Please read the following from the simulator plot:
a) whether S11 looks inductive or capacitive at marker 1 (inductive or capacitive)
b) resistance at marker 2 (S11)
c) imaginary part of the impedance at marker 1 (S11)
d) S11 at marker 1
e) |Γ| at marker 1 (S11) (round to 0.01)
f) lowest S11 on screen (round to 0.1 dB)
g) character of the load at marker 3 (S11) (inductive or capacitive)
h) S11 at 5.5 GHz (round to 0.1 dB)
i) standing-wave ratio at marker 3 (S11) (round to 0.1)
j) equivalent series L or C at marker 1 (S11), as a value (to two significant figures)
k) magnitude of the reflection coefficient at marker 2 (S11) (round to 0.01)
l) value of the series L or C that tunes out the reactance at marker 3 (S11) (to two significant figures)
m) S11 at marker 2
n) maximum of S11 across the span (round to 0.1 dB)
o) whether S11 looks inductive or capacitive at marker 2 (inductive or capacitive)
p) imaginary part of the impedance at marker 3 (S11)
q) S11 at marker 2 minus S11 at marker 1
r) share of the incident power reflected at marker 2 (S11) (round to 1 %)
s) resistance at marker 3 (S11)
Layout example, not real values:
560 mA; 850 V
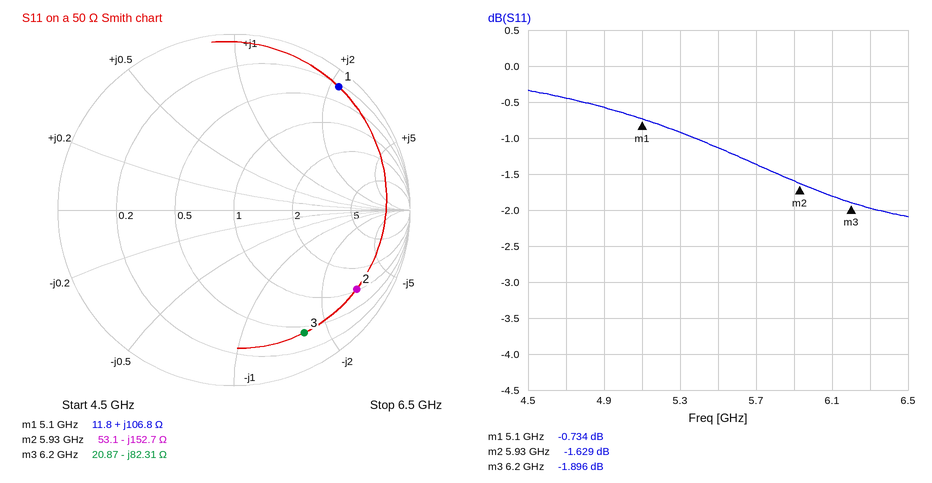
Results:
inductive; 53.1 Ω; +106.8 Ω; -0.734 dB; 0.92; -2.1 dB; capacitive; -1.1 dB; 9.2; 3.3 nH; 0.83; 2.1 nH; -1.629 dB; -0.3 dB; capacitive; -82.31 Ω; -0.895 dB; 69 %; 20.87 Ω
